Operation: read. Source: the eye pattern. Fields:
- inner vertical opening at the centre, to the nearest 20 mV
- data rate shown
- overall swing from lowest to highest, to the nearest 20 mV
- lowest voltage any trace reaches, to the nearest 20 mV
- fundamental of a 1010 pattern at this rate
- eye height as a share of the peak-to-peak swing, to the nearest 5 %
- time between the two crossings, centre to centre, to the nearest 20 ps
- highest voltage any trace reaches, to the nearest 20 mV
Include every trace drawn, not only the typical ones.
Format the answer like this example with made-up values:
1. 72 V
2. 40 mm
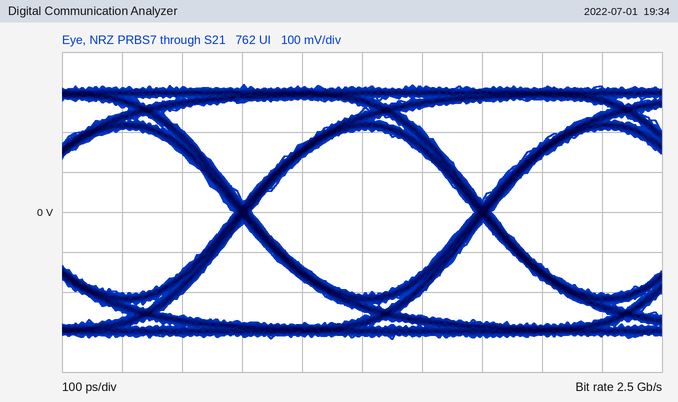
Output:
1. 420 mV
2. 2.5 Gb/s
3. 640 mV
4. -320 mV
5. 1.25 GHz
6. 65 %
7. 400 ps
8. 320 mV
